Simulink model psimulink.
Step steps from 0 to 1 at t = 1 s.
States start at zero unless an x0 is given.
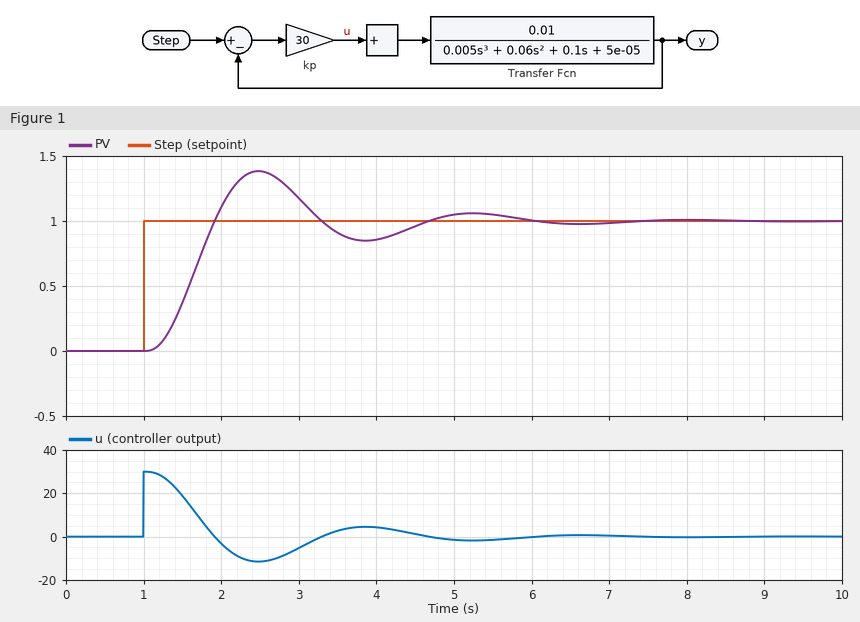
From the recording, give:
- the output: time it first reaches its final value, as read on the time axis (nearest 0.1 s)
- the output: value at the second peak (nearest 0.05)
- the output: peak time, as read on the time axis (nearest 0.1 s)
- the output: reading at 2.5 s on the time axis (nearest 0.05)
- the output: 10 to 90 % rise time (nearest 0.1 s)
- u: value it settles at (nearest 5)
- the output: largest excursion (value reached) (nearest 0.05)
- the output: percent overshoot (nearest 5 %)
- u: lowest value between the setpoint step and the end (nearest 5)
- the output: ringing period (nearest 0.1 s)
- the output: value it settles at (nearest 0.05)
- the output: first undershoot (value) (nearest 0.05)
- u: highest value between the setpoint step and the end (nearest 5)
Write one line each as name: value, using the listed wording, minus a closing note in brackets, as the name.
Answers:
the output: time it first reaches its final value, as read on the time axis: 1.9 s
the output: value at the second peak: 1.05
the output: peak time, as read on the time axis: 2.5 s
the output: reading at 2.5 s on the time axis: 1.40
the output: 10 to 90 % rise time: 0.6 s
u: value it settles at: 0
the output: largest excursion (value reached): 1.40
the output: percent overshoot: 40 %
u: lowest value between the setpoint step and the end: -10
the output: ringing period: 2.8 s
the output: value it settles at: 1.00
the output: first undershoot (value): 0.85
u: highest value between the setpoint step and the end: 30
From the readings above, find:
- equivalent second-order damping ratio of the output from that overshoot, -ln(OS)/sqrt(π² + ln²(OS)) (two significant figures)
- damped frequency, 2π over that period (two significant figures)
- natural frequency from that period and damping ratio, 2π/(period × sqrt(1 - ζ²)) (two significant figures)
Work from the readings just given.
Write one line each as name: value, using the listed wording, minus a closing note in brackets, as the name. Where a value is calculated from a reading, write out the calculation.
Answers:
equivalent second-order damping ratio of the output from that overshoot, -ln(OS)/sqrt(π² + ln²(OS)): ln(0.4) = -0.916; 0.916 / sqrt(9.870 + 0.840) = 0.28
damped frequency, 2π over that period: 2π / 2.8 = 2.2 rad/s
natural frequency from that period and damping ratio, 2π/(period × sqrt(1 - ζ²)): 2π / (2.8 × sqrt(1 - 0.28²)) = 2.3 rad/s
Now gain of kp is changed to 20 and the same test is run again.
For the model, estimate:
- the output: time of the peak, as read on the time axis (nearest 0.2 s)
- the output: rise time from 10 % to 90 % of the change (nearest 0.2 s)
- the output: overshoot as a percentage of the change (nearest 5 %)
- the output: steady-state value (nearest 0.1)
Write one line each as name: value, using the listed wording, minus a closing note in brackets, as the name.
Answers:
the output: time of the peak, as read on the time axis: 2.8 s
the output: rise time from 10 % to 90 % of the change: 0.8 s
the output: overshoot as a percentage of the change: 25 %
the output: steady-state value: 1.0
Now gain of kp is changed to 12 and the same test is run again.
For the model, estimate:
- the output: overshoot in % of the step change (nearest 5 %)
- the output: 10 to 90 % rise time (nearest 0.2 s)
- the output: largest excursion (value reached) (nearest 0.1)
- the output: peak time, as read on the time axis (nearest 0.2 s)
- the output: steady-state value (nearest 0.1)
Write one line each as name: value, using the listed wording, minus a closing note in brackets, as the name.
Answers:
the output: overshoot in % of the step change: 10 %
the output: 10 to 90 % rise time: 1.2 s
the output: largest excursion (value reached): 1.1
the output: peak time, as read on the time axis: 3.6 s
the output: steady-state value: 1.0
